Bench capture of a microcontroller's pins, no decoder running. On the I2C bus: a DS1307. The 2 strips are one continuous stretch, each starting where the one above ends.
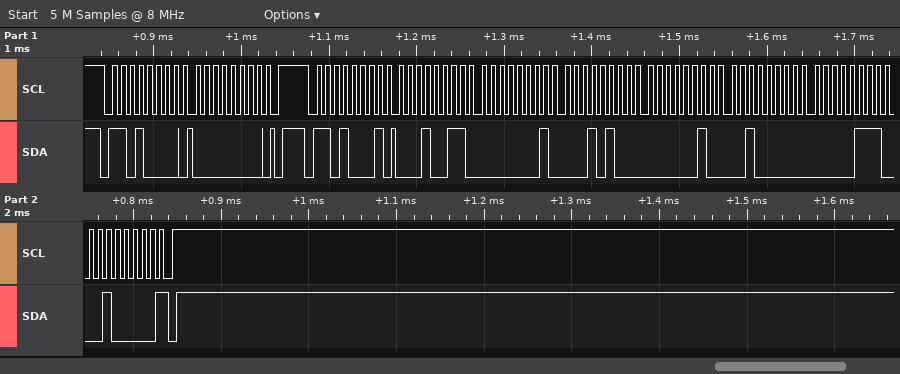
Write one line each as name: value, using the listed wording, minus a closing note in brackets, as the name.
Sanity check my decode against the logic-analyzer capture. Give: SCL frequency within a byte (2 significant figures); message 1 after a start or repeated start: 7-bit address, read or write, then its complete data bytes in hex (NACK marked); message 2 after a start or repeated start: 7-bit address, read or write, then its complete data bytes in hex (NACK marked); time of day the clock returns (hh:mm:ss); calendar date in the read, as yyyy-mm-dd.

SCL frequency within a byte: 100 kHz
message 1 after a start or repeated start: 7-bit address, read or write, then its complete data bytes in hex: 0x68 write: 00
message 2 after a start or repeated start: 7-bit address, read or write, then its complete data bytes in hex: 0x68 read: 13 01 14 02 20 07 20 NACK
time of day the clock returns: 14:01:13
calendar date in the read, as yyyy-mm-dd: 2020-07-20
